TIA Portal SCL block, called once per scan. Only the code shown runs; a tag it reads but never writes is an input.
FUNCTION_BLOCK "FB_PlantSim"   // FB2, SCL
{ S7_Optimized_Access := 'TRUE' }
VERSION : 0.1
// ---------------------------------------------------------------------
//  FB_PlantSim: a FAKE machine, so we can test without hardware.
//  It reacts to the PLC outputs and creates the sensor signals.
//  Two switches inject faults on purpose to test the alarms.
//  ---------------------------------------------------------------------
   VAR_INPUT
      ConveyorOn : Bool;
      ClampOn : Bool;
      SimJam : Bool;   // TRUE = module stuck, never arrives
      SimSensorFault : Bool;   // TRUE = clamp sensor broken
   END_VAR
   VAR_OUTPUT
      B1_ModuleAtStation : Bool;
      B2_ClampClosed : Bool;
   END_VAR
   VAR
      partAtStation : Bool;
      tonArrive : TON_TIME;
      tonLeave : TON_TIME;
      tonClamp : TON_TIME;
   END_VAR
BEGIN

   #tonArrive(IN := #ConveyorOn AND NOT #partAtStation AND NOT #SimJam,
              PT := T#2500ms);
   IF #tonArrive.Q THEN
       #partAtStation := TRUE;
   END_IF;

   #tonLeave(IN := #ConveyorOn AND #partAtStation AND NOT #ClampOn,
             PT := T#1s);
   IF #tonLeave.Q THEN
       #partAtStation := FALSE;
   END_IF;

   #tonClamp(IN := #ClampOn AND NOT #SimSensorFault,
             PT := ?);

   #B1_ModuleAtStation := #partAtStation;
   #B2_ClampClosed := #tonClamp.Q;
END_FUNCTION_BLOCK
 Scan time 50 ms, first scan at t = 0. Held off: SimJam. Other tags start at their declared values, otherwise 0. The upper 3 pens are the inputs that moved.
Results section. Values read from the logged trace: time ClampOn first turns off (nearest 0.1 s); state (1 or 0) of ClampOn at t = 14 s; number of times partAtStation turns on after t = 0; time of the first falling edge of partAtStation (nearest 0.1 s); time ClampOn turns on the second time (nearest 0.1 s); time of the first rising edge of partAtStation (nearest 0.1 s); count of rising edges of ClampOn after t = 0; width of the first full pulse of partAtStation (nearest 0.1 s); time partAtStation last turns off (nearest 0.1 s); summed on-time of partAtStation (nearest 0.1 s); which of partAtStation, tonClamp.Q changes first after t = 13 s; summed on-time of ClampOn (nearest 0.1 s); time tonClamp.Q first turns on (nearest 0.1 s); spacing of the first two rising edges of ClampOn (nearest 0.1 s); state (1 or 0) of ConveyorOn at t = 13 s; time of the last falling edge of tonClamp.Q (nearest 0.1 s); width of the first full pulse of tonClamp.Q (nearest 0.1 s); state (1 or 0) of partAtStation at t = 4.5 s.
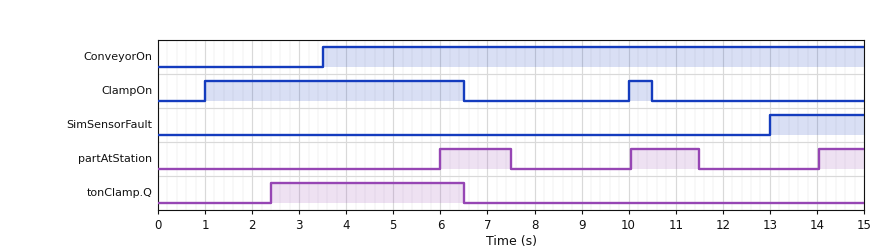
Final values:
6.5 s
0
3
7.5 s
10.0 s
6.0 s
2
1.5 s
11.5 s
3.9 s
partAtStation
6.0 s
2.4 s
9.0 s
1
6.5 s
4.1 s
0
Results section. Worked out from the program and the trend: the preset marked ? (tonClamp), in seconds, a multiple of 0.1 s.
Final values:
1.4 s
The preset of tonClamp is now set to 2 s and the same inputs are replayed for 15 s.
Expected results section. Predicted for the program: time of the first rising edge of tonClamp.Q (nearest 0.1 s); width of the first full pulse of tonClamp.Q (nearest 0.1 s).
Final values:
3.0 s
3.5 s
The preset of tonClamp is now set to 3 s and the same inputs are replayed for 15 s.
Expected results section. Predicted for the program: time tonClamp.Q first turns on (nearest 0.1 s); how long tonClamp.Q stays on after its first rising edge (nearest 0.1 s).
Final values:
4.0 s
2.5 s
